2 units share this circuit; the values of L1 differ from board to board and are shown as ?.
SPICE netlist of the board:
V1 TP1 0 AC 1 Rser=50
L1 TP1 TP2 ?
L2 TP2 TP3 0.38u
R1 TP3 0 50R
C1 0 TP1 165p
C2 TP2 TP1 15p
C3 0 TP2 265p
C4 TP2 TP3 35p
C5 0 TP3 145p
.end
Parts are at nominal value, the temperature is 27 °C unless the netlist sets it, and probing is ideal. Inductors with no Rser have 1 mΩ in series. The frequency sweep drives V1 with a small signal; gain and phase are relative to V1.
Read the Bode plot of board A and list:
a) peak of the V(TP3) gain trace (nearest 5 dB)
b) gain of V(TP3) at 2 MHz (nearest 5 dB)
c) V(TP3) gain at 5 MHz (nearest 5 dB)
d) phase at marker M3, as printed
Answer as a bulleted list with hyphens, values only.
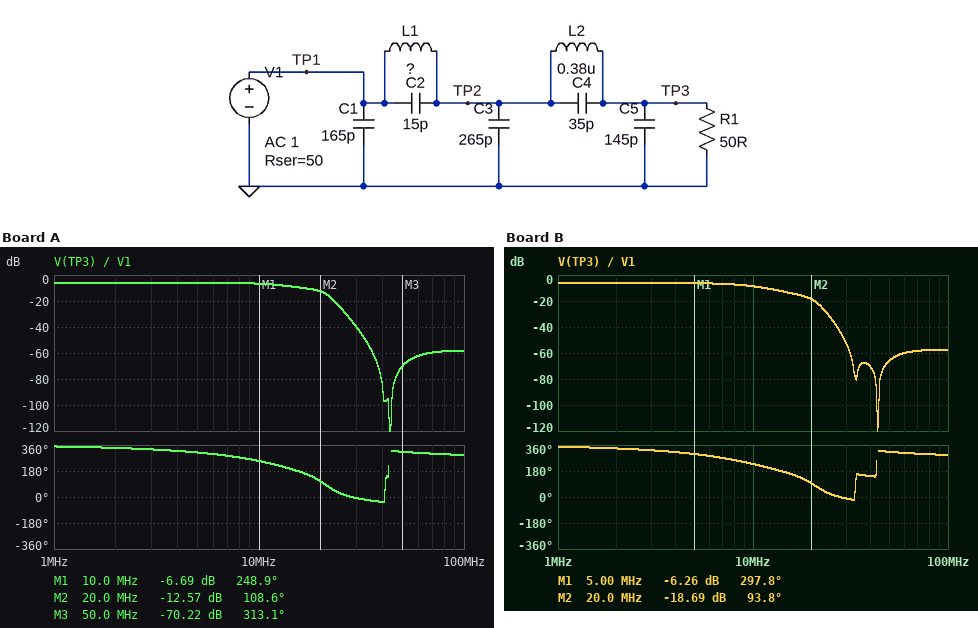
- -5 dB
- -5 dB
- -5 dB
- 313.1 deg
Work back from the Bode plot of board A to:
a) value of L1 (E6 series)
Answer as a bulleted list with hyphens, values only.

- 1 µH
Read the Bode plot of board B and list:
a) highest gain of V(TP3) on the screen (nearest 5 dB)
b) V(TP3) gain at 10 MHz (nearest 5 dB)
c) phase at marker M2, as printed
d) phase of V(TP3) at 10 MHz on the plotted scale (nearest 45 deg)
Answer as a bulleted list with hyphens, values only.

- -5 dB
- -10 dB
- 93.8 deg
- 225 deg
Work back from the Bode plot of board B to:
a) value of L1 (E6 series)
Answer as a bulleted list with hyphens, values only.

- 1.5 µH
